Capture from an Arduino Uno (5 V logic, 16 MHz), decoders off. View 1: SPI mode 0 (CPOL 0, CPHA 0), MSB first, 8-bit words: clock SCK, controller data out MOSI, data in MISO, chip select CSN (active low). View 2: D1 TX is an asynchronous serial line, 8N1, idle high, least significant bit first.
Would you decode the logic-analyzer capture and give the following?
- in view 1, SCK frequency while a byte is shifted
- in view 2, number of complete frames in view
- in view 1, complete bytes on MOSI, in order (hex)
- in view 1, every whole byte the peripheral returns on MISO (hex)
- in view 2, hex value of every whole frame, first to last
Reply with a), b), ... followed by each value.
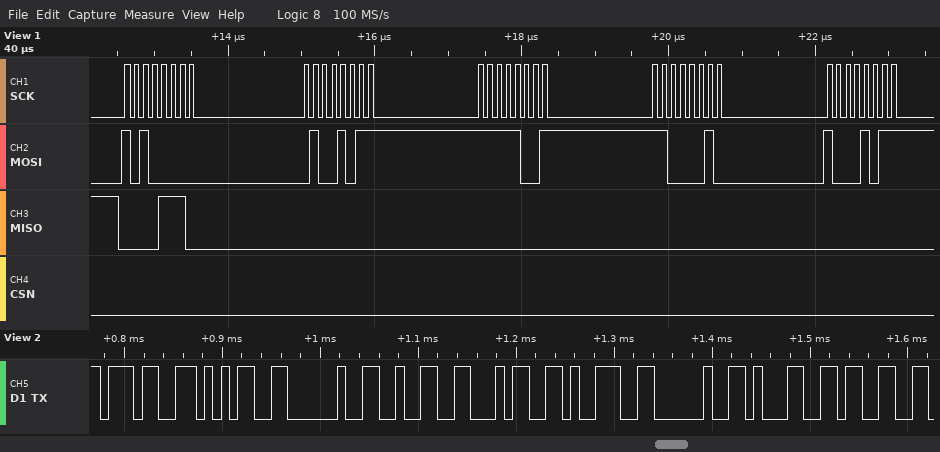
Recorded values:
a) 8 MHz
b) 9
c) A0 4B F9 C2 8B
d) 0E 00 00 00 00
e) 37 35 20 32 34 39 20 31 33
